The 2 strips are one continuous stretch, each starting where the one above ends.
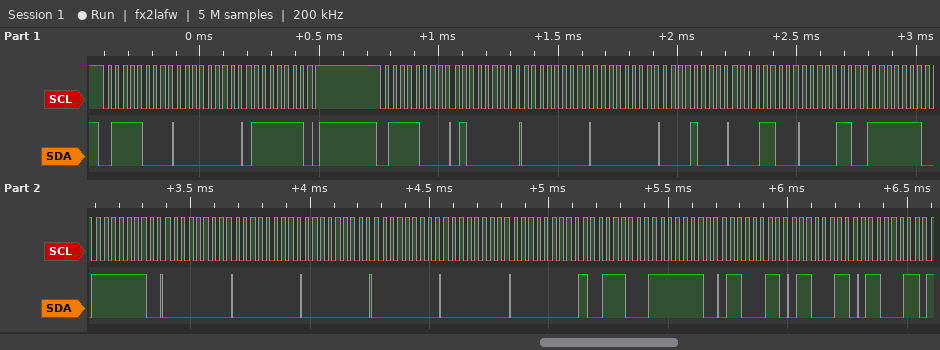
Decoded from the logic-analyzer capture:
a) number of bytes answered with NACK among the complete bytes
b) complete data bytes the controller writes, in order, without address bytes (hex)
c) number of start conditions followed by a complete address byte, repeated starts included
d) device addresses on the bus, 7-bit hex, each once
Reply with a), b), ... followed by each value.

a) 0
b) 00 7F 40 00 00 08 0C 06 FE FE 00 00 00 00 00 00 9C FE 63 63 63
c) 2
d) 0x3C
